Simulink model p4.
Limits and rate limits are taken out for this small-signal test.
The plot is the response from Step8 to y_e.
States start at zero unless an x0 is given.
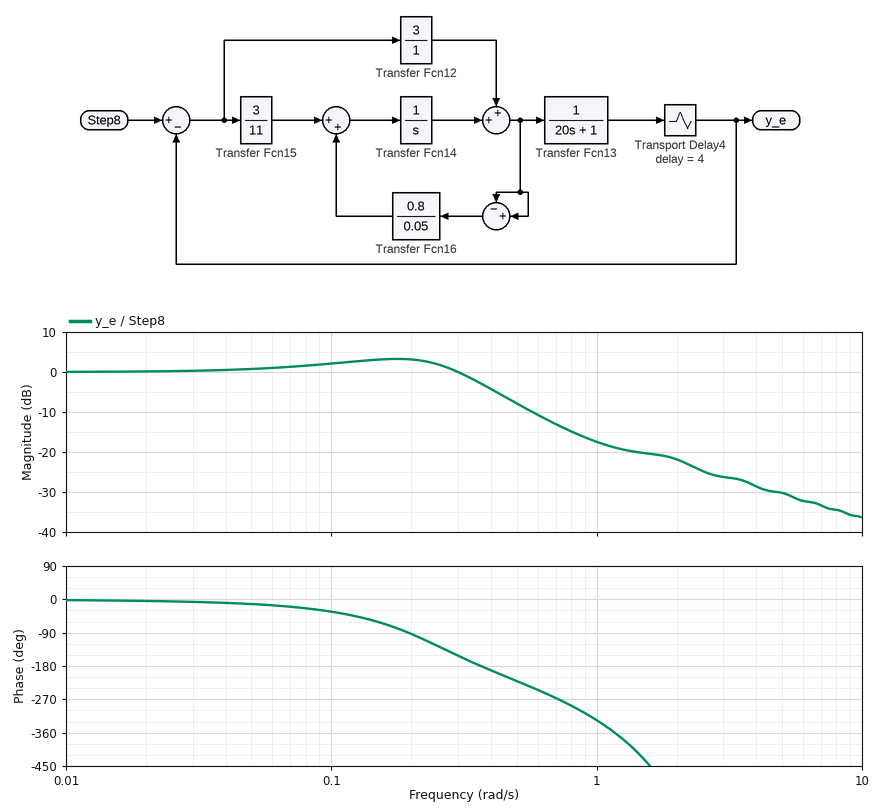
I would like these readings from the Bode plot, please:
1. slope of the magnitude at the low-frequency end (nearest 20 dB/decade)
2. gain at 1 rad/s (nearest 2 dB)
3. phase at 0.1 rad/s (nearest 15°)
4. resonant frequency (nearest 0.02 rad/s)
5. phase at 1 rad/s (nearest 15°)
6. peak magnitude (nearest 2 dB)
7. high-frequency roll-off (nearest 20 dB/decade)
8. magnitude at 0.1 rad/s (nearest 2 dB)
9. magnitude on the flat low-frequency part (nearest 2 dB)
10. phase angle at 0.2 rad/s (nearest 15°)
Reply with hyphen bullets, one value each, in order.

- 0 dB/decade
- -18 dB
- -30°
- 0.18 rad/s
- -330°
- 4 dB
- -20 dB/decade
- 2 dB
- 0 dB
- -90°
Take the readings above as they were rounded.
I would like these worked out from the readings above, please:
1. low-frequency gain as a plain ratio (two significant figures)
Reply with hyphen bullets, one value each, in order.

- 1.0
